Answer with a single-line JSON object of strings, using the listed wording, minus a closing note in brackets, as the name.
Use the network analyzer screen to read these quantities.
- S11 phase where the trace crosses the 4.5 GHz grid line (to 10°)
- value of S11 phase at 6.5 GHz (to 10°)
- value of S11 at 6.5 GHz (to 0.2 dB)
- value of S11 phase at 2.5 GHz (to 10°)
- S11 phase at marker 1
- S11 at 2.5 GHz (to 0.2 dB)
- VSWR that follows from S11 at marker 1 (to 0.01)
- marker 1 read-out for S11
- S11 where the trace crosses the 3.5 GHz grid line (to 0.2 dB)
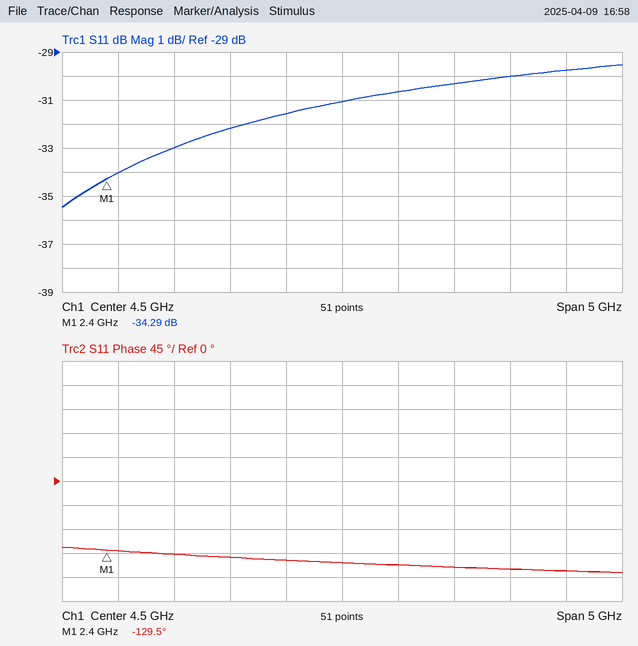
{"S11 phase where the trace crosses the 4.5 GHz grid line": "-150°", "value of S11 phase at 6.5 GHz": "-170°", "value of S11 at 6.5 GHz": "-29.8 dB", "value of S11 phase at 2.5 GHz": "-130°", "S11 phase at marker 1": "-129.5°", "S11 at 2.5 GHz": "-34.0 dB", "VSWR that follows from S11 at marker 1": "1.04", "marker 1 read-out for S11": "-34.29 dB", "S11 where the trace crosses the 3.5 GHz grid line": "-32.2 dB"}
